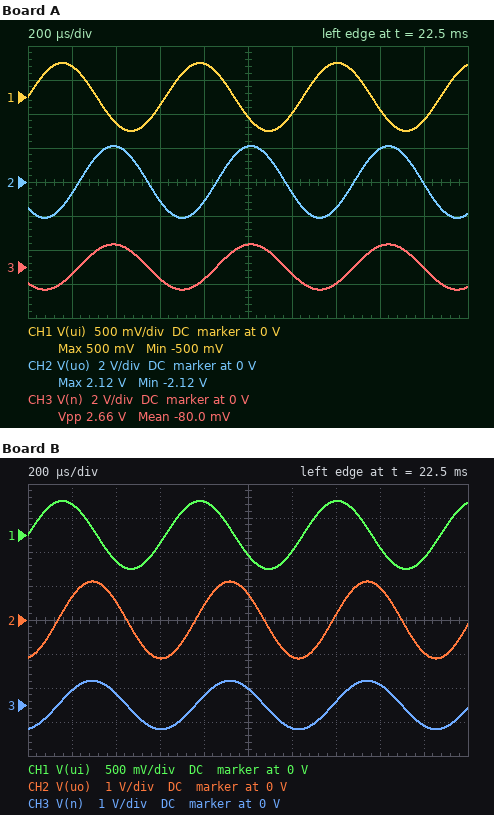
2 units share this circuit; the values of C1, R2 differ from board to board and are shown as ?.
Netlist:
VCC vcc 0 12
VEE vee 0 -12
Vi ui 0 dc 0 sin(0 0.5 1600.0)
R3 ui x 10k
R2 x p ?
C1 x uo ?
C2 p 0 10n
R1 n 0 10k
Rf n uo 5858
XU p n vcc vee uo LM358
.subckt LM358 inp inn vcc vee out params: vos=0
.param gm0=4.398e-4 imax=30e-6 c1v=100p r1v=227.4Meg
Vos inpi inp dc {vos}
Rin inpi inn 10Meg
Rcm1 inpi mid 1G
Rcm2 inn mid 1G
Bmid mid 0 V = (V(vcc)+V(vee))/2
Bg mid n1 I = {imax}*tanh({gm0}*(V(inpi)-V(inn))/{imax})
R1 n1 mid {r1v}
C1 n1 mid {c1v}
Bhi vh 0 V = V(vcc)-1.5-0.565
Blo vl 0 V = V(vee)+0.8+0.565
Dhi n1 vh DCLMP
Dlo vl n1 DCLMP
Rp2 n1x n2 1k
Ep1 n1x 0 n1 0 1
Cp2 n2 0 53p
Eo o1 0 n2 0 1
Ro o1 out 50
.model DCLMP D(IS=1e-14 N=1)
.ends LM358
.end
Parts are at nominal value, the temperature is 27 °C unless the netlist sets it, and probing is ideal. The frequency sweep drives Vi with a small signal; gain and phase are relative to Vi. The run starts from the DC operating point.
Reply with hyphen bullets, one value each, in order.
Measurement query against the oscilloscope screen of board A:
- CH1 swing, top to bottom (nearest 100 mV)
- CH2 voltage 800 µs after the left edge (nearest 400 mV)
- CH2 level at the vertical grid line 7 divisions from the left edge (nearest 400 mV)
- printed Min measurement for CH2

- 1.0 V
- -1.2 V
- -1.6 V
- -2.12 V
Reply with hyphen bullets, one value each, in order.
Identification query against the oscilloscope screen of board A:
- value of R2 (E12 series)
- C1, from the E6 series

- 5.6 kΩ
- 22 nF
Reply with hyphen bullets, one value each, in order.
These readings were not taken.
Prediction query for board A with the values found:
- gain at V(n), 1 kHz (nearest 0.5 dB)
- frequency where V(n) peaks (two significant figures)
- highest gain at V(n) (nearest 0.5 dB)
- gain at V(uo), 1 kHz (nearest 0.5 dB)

- 5.5 dB
- 1.4 kHz
- 12.5 dB
- 9.5 dB
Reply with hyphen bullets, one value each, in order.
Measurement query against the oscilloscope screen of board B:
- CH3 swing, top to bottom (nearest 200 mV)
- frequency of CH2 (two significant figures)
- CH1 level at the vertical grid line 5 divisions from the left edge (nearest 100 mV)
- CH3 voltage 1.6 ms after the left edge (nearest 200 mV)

- 1.4 V
- 1.6 kHz
- -300 mV
- 600 mV
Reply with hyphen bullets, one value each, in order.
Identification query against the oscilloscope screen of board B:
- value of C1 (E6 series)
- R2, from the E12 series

- 15 nF
- 5.6 kΩ
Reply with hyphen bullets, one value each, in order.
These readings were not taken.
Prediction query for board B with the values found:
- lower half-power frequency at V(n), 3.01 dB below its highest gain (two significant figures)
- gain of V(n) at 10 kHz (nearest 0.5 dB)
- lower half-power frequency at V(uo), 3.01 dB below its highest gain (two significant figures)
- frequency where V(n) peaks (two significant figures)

- 340 Hz
- -30.5 dB
- 340 Hz
- 1.5 kHz
